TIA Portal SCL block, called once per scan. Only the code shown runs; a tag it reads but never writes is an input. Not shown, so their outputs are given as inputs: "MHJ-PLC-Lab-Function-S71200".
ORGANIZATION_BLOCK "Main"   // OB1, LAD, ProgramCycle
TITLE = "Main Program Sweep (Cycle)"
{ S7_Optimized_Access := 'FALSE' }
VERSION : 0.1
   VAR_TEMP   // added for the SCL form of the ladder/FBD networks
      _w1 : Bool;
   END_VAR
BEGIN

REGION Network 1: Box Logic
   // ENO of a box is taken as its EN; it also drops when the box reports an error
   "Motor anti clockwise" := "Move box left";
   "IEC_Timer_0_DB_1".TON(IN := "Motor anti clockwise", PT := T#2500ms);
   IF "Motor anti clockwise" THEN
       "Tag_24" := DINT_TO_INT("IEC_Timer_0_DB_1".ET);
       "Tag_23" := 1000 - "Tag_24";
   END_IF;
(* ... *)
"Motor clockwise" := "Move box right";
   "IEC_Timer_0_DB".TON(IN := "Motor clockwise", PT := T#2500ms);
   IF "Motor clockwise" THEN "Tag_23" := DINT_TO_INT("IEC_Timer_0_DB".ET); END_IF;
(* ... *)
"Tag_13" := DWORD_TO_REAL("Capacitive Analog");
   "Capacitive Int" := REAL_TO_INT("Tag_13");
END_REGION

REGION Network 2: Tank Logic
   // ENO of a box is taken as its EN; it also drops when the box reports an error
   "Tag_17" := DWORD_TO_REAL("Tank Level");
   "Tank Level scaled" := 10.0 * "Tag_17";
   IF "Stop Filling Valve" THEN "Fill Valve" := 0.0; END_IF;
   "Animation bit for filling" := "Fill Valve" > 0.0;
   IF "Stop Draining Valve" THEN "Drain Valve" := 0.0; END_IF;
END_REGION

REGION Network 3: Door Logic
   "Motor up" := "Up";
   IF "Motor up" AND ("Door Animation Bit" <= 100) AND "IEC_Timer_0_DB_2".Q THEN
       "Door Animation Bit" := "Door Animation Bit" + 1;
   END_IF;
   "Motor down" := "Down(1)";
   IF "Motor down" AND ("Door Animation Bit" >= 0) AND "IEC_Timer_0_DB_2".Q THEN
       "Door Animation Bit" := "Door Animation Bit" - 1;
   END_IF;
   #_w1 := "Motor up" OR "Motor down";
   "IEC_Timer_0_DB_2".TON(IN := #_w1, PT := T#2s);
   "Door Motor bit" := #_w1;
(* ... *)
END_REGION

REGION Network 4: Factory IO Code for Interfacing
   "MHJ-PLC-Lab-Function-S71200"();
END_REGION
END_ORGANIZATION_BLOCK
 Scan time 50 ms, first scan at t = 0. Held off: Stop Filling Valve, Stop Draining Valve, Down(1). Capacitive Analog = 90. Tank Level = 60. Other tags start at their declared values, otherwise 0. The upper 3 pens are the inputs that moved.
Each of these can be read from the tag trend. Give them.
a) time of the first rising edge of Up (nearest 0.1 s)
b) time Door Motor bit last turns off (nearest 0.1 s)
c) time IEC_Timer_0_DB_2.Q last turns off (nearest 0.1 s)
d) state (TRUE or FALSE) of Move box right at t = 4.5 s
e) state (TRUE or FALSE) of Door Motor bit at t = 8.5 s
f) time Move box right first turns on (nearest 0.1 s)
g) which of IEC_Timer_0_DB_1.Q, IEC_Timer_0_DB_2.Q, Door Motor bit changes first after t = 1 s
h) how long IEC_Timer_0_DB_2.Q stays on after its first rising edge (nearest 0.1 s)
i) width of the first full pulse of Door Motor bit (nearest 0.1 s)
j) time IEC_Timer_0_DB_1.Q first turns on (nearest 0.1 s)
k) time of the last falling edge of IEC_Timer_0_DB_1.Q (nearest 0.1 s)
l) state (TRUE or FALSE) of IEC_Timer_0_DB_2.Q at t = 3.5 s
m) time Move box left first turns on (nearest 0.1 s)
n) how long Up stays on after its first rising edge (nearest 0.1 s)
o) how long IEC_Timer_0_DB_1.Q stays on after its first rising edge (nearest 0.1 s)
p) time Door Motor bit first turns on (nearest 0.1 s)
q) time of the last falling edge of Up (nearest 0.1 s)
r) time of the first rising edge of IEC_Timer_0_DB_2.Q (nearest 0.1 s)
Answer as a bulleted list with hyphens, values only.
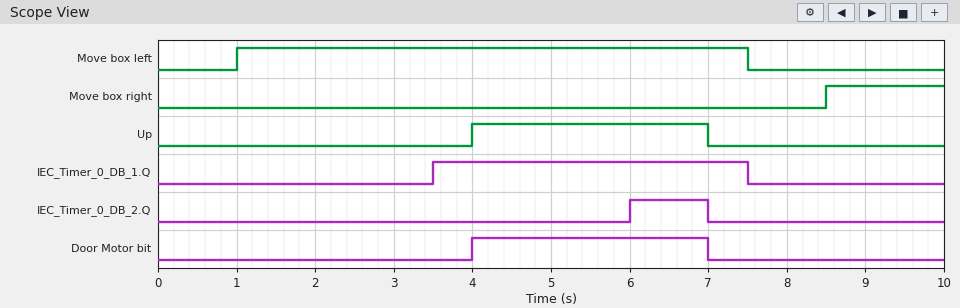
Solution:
- 4.0 s
- 7.0 s
- 7.0 s
- FALSE
- FALSE
- 8.5 s
- IEC_Timer_0_DB_1.Q
- 1.0 s
- 3.0 s
- 3.5 s
- 7.5 s
- FALSE
- 1.0 s
- 3.0 s
- 4.0 s
- 4.0 s
- 7.0 s
- 6.0 s
